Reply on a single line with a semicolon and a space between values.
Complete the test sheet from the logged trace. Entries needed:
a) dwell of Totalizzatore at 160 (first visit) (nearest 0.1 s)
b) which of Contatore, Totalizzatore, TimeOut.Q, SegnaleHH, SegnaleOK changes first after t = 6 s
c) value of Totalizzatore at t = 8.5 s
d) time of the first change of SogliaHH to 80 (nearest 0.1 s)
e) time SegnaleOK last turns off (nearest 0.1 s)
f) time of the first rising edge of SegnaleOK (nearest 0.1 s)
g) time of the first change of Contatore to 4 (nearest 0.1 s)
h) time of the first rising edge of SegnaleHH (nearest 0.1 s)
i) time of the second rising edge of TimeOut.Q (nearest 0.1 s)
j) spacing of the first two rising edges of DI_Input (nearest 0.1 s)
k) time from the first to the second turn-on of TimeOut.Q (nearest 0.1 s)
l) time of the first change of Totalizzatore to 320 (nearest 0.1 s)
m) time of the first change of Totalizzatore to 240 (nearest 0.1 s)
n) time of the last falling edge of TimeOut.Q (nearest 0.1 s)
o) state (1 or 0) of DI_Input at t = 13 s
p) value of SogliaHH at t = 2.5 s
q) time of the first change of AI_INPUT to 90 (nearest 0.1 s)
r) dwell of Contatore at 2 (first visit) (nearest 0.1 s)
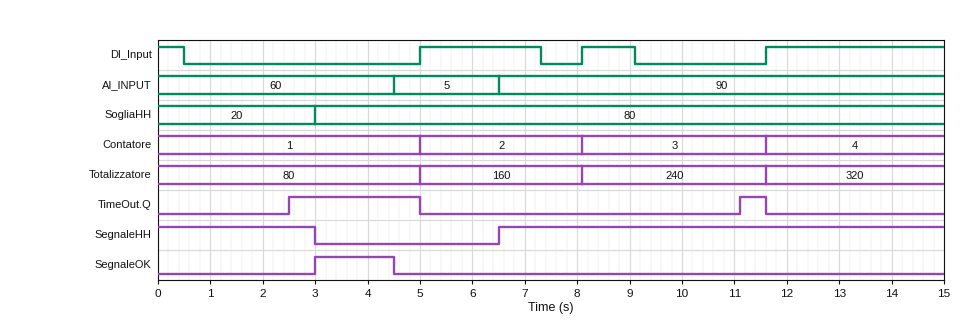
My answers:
3.1 s; SegnaleHH; 240; 3.0 s; 4.5 s; 3.0 s; 11.6 s; 6.5 s; 11.1 s; 3.1 s; 8.6 s; 11.6 s; 8.1 s; 11.6 s; 1; 20; 6.5 s; 3.1 s
